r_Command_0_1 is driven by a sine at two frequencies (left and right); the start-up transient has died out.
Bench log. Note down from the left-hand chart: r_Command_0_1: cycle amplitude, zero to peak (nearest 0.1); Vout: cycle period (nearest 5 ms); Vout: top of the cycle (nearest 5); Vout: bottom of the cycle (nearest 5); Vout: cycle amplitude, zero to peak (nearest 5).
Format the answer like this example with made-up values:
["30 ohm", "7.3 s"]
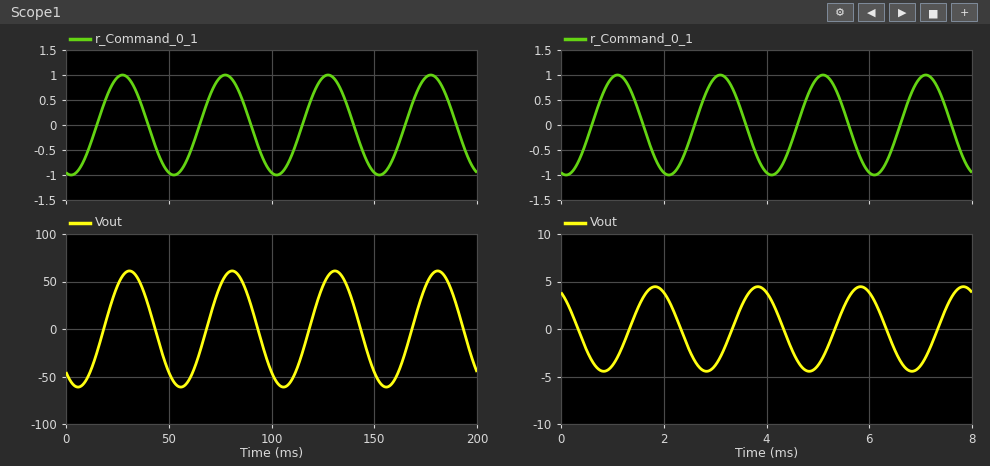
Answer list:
["1.0", "50 ms", "60", "-60", "60"]
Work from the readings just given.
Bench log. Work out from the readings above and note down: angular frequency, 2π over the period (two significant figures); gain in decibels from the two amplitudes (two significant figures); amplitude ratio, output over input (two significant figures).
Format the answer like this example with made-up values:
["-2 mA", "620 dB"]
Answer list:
["0.13 rad/ms", "36 dB", "60"]
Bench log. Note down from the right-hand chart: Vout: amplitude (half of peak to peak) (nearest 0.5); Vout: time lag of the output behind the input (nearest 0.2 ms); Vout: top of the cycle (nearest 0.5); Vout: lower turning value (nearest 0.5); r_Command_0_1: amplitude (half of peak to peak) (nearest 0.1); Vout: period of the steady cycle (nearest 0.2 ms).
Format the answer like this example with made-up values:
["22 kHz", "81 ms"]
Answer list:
["4.5", "0.8 ms", "4.5", "-4.5", "1.0", "2.0 ms"]
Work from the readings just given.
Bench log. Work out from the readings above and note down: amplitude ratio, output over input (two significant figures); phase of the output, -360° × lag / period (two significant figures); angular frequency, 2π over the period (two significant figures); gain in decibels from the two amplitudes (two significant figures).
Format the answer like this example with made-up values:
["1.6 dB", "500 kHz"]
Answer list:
["4.5", "-140°", "3.1 rad/ms", "13 dB"]
